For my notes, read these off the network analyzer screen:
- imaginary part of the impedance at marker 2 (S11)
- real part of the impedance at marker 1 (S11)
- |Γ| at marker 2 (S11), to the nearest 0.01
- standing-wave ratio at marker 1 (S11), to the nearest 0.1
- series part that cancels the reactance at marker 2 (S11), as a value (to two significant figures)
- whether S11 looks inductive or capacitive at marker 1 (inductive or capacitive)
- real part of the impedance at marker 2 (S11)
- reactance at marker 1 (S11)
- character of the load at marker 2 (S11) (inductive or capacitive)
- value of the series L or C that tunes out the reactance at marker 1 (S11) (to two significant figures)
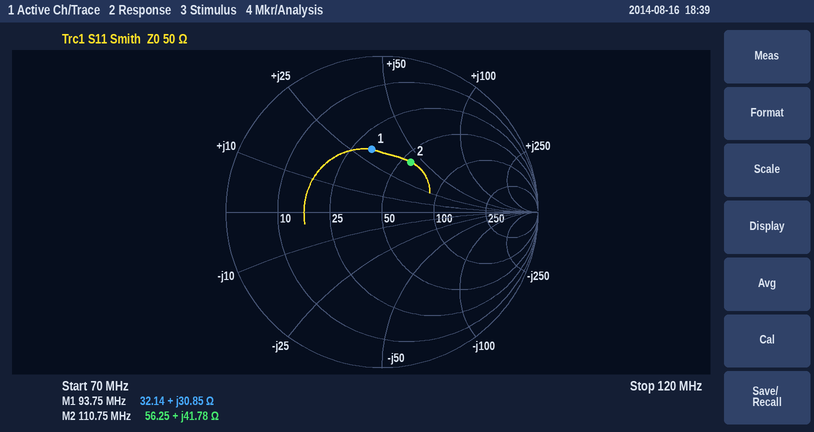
+41.78 Ω
32.14 Ω
0.37
2.4
34 pF
inductive
56.25 Ω
+30.85 Ω
inductive
55 pF
